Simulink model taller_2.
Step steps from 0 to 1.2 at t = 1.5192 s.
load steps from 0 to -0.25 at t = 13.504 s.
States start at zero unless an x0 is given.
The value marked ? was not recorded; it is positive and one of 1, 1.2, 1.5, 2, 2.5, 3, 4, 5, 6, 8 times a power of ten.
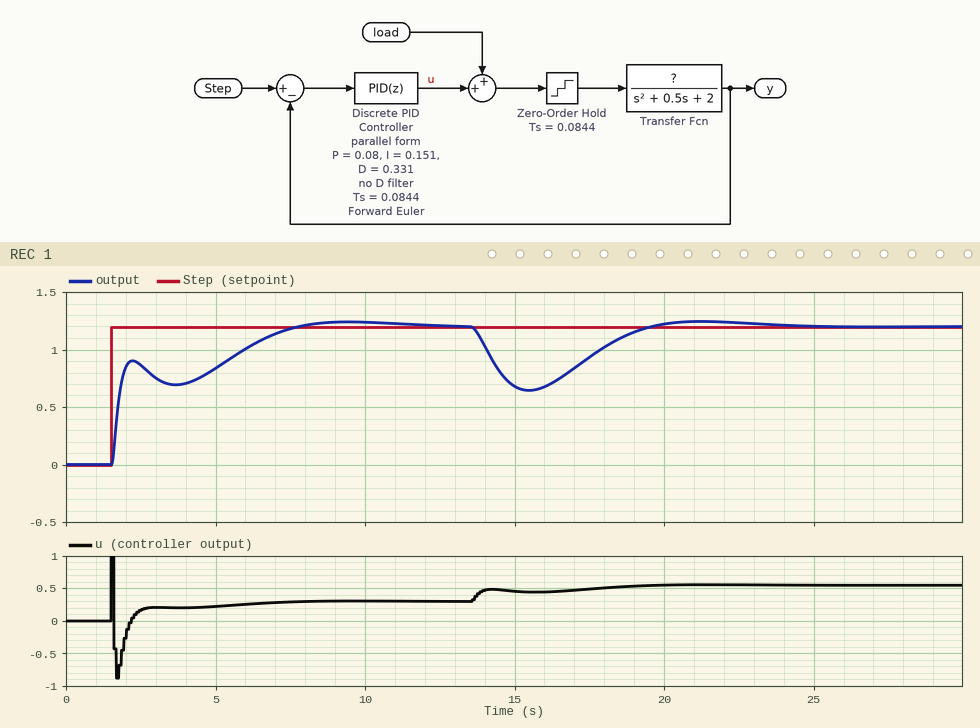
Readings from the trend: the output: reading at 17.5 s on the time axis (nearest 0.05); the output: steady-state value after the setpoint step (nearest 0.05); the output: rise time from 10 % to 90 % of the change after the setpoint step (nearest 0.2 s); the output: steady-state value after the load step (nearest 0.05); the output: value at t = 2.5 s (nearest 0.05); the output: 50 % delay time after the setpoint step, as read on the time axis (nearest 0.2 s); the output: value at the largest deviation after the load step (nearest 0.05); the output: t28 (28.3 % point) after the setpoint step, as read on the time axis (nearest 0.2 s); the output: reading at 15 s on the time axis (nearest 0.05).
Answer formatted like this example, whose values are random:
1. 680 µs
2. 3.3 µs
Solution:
1. 0.95
2. 1.20
3. 5.0 s
4. 1.20
5. 0.85
6. 1.8 s
7. 0.65
8. 1.6 s
9. 0.70
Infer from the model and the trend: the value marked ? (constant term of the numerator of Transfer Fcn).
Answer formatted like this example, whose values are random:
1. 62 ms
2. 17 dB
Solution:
1. 8
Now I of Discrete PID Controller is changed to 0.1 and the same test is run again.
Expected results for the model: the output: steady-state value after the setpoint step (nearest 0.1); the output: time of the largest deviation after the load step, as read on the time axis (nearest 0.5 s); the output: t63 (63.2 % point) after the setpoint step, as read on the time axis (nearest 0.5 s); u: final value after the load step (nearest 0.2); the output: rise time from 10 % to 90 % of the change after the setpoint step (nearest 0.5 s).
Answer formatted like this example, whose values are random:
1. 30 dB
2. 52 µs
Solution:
1. 1.2
2. 15.5 s
3. 2.0 s
4. 0.6
5. 6.5 s
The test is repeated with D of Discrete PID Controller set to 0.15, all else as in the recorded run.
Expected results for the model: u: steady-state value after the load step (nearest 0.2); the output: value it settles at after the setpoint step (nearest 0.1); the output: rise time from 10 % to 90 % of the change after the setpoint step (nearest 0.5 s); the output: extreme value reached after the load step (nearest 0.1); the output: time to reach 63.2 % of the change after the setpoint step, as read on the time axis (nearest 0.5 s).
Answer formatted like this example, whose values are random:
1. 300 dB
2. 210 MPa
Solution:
1. 0.6
2. 1.2
3. 4.0 s
4. 0.5
5. 2.5 s
